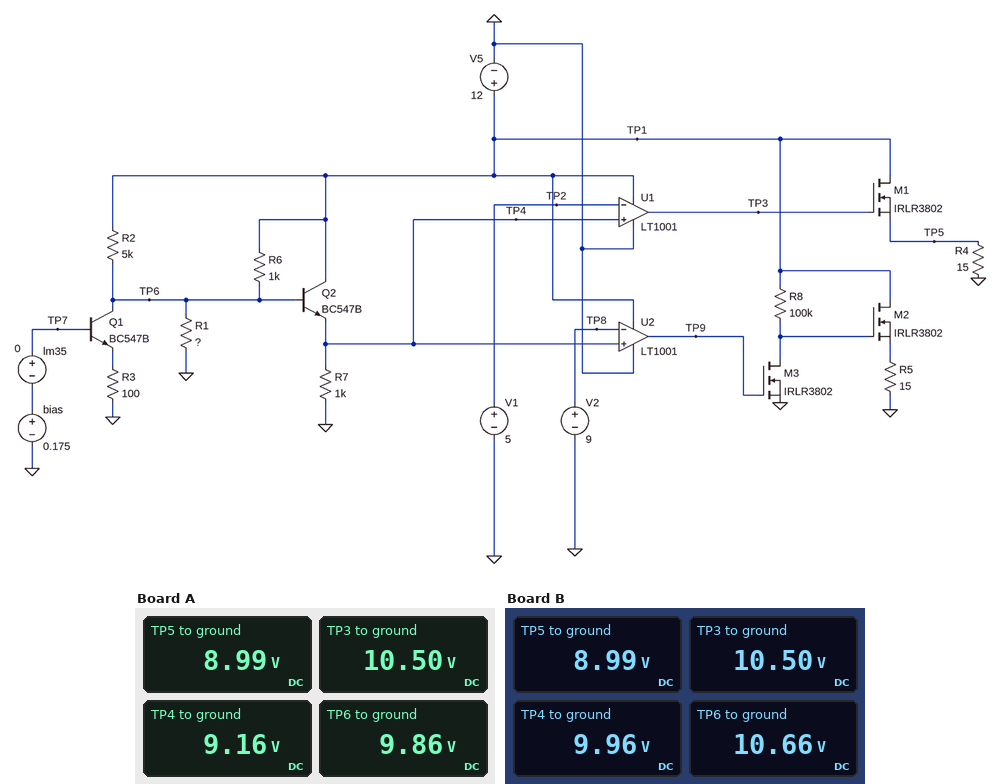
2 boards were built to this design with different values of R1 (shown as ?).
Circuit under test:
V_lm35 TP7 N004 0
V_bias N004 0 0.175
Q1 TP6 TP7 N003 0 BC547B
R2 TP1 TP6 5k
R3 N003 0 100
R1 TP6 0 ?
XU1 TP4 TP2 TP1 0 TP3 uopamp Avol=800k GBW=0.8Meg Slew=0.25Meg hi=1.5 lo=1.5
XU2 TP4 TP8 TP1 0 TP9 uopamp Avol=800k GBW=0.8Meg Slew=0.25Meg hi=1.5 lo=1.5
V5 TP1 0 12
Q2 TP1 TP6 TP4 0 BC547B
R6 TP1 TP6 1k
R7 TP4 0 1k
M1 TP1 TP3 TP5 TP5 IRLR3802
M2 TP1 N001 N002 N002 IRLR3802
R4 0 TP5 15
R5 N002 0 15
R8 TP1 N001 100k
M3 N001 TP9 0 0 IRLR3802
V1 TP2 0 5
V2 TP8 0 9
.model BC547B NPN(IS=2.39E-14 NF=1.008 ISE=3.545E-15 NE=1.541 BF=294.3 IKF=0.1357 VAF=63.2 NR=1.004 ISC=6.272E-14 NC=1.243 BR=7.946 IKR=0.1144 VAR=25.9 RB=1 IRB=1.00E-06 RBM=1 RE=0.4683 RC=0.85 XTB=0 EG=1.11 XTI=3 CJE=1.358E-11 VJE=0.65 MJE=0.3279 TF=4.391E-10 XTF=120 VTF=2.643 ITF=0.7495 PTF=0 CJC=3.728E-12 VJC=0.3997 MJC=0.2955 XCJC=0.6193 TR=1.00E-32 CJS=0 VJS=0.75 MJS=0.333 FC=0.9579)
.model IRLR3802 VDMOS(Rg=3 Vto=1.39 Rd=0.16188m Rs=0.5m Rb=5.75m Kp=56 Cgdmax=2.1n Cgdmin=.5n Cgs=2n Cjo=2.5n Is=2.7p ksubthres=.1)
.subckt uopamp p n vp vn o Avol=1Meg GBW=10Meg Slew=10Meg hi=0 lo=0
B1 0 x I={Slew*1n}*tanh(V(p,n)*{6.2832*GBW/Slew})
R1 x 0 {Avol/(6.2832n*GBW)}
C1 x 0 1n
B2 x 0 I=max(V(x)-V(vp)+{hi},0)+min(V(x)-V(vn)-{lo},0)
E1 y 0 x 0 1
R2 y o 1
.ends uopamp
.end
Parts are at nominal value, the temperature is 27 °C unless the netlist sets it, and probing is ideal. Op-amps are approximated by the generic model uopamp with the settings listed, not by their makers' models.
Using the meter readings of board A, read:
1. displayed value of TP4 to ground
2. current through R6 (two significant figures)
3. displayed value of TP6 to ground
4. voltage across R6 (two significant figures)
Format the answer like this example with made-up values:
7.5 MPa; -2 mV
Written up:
9.16 V; 2.1 mA; 9.86 V; 2.1 V
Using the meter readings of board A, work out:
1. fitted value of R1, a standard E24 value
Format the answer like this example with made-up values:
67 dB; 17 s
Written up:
3.9 kΩ
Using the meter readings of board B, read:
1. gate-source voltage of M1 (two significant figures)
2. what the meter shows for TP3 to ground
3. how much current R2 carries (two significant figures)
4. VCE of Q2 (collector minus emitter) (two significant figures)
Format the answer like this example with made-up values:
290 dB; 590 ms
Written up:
1.5 V; 10.50 V; 270 µA; 2.0 V
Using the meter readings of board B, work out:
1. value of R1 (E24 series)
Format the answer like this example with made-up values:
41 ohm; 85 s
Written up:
6.8 kΩ
